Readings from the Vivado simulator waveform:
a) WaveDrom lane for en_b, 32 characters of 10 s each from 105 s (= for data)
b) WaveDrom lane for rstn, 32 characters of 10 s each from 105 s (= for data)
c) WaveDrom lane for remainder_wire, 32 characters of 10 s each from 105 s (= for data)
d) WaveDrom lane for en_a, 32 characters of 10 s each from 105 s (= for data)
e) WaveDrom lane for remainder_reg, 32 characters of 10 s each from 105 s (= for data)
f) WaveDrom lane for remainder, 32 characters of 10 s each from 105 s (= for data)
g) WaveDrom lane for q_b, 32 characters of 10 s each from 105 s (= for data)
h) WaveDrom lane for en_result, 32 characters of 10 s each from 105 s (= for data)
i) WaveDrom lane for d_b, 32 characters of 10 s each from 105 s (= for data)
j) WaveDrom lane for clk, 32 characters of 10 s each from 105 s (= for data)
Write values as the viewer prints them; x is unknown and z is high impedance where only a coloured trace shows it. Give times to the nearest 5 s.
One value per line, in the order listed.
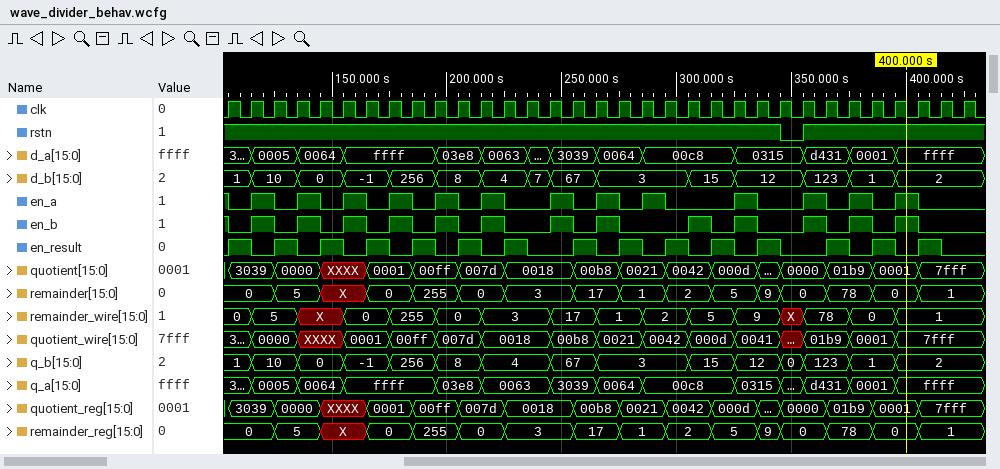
{name: 'en_b', wave: '0101010101010.1010..1010.101010.'}
{name: 'rstn', wave: '1.......................01......'}
{name: 'remainder_wire', wave: '==.x.=.=.=.=..=.=.=.=.=.x=.=.=..', data: '0 5 0 255 0 3 17 1 2 5 9 78 0 1'}
{name: 'en_a', wave: '0101010101010.101010..10.101010.'}
{name: 'remainder_reg', wave: '=.=.x.=.=.=.=..=.=.=.=.==.=.=.=.', data: '0 5 0 255 0 3 17 1 2 5 9 0 78 0 1'}
{name: 'remainder', wave: '=.=.x.=.=.=.=..=.=.=.=.==.=.=.=.', data: '0 5 0 255 0 3 17 1 2 5 9 0 78 0 1'}
{name: 'q_b', wave: '==.=.=.=.=.=..=.=...=.=.==.=.=..', data: '1 10 0 -1 256 8 4 67 3 15 12 0 123 1 2'}
{name: 'en_result', wave: '10101010101010.1010101010.101010'}
{name: 'd_b', wave: '==.=.=.=.=.=.==.=...=.=..=.=.=..', data: '1 10 0 -1 256 8 4 7 67 3 15 12 123 1 2'}
{name: 'clk', wave: 'p...............................'}
